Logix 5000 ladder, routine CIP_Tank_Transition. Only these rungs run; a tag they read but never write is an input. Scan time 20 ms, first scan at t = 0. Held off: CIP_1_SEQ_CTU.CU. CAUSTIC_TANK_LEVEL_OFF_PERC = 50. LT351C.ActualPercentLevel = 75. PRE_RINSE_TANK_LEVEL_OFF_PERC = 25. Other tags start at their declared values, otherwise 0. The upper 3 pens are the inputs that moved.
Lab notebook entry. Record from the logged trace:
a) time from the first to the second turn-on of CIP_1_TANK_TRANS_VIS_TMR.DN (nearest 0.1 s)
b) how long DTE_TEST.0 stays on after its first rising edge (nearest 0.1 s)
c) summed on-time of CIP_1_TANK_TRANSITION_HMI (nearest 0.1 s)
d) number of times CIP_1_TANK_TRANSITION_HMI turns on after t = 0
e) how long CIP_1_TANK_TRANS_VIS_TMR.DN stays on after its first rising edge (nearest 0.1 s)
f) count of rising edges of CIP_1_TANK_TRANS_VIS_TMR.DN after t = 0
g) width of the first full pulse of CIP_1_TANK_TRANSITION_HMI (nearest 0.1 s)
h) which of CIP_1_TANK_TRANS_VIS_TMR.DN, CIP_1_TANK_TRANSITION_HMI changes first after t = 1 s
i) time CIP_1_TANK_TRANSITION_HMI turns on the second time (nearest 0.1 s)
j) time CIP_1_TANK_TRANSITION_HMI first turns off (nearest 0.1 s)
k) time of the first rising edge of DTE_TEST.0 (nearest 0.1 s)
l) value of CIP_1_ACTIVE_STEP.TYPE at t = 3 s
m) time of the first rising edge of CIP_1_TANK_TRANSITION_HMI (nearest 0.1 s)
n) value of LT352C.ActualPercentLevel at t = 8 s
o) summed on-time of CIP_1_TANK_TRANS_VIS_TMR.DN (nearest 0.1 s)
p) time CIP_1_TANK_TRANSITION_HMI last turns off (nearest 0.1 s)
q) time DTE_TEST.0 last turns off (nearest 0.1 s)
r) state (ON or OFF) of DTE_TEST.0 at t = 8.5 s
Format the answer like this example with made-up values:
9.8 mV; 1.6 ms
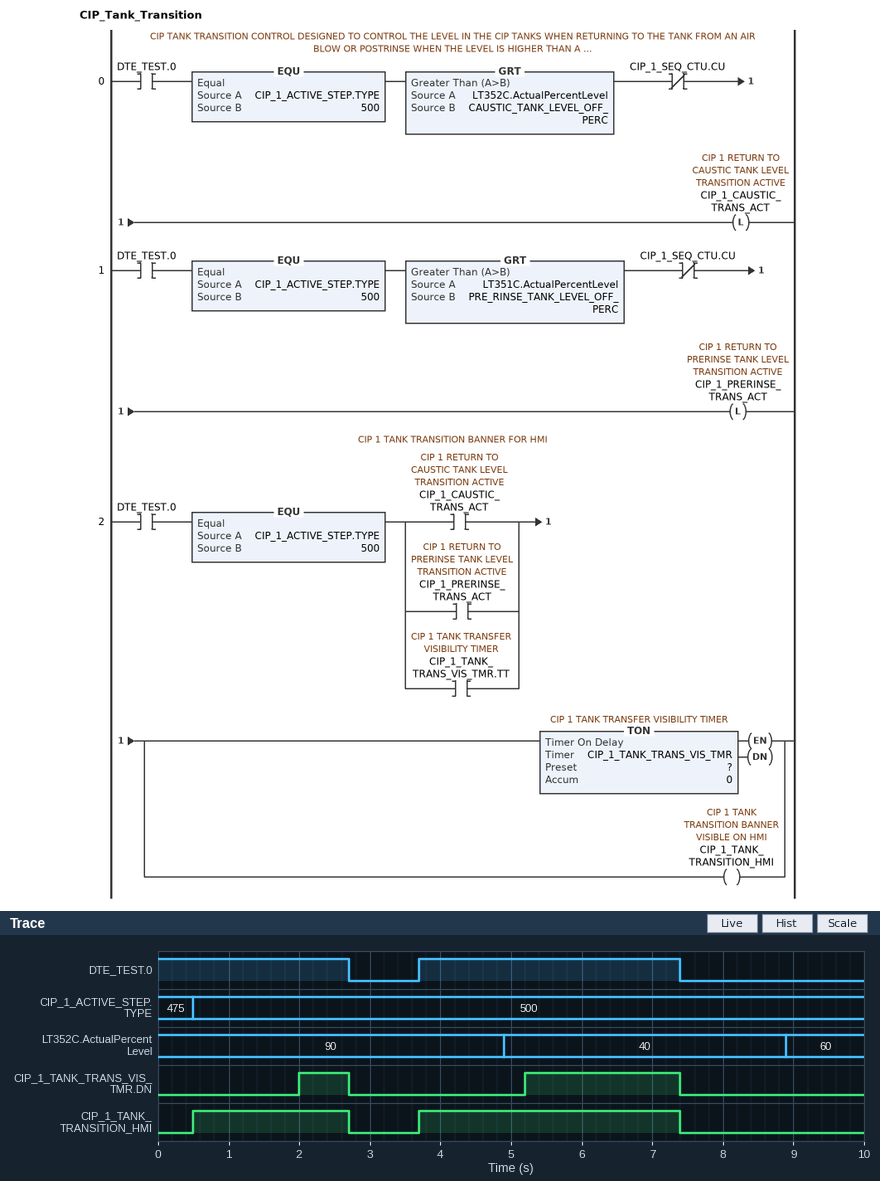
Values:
3.2 s; 3.7 s; 5.9 s; 2; 0.7 s; 2; 2.2 s; CIP_1_TANK_TRANS_VIS_TMR.DN; 3.7 s; 2.7 s; 3.7 s; 500; 0.5 s; 40; 2.9 s; 7.4 s; 7.4 s; OFF
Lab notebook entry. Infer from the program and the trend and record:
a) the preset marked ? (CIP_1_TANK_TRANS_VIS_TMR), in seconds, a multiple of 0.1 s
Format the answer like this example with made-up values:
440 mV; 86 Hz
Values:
1.5 s
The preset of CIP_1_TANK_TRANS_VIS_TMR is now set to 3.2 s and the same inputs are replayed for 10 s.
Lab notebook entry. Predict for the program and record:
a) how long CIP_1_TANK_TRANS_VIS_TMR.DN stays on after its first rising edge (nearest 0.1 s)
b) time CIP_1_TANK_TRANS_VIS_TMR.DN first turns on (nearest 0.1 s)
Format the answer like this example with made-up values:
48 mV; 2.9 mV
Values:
0.5 s; 6.9 s
